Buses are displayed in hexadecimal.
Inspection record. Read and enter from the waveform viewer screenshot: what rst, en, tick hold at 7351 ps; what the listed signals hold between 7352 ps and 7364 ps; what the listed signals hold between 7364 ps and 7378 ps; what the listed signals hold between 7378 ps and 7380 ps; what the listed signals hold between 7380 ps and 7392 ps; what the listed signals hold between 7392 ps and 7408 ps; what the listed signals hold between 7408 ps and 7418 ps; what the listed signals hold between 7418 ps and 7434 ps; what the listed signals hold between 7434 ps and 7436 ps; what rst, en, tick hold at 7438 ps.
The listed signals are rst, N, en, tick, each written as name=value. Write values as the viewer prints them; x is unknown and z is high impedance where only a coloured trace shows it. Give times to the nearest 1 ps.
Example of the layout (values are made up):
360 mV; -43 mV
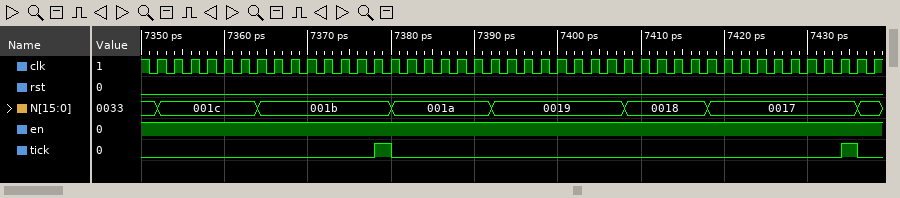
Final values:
rst=0, en=1, tick=0; rst=0, N=001c, en=1, tick=0; rst=0, N=001b, en=1, tick=0; rst=0, N=001b, en=1, tick=1; rst=0, N=001a, en=1, tick=0; rst=0, N=0019, en=1, tick=0; rst=0, N=0018, en=1, tick=0; rst=0, N=0017, en=1, tick=0; rst=0, N=0017, en=1, tick=1; rst=0, en=1, tick=0
